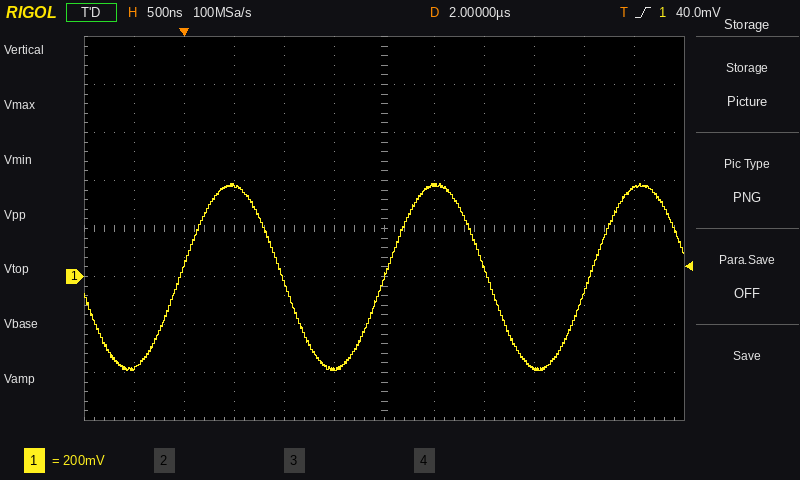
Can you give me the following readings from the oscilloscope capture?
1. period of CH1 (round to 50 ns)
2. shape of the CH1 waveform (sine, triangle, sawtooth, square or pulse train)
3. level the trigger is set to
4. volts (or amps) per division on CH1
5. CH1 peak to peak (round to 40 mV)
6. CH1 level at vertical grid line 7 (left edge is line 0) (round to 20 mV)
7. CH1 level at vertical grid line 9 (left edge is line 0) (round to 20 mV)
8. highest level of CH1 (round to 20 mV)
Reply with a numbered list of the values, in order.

1. 2.05 µs
2. sine
3. 40.0 mV
4. 200 mV
5. 760 mV
6. 380 mV
7. -380 mV
8. 380 mV
